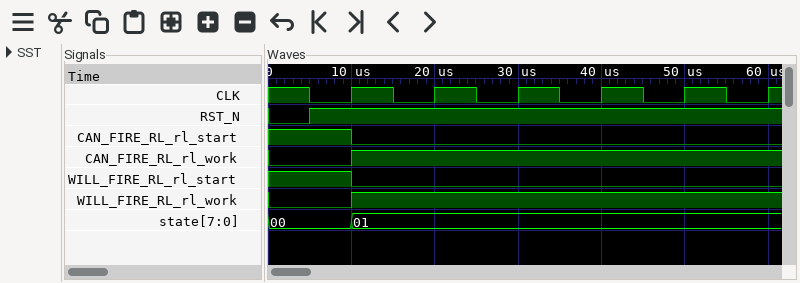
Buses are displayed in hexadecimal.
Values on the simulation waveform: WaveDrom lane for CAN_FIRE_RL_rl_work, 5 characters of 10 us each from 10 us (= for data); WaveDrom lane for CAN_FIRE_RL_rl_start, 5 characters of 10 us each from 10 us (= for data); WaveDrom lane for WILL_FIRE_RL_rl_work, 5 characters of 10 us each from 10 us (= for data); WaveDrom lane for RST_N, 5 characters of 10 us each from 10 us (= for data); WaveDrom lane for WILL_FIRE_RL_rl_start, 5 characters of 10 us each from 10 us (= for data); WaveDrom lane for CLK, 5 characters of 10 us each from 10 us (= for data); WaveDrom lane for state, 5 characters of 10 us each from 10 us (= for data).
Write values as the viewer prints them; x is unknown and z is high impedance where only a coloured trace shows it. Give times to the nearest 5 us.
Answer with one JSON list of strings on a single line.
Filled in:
["{name: 'CAN_FIRE_RL_rl_work', wave: '1....'}", "{name: 'CAN_FIRE_RL_rl_start', wave: '0....'}", "{name: 'WILL_FIRE_RL_rl_work', wave: '1....'}", "{name: 'RST_N', wave: '1....'}", "{name: 'WILL_FIRE_RL_rl_start', wave: '0....'}", "{name: 'CLK', wave: 'p....'}", "{name: 'state', wave: '=....', data: '01'}"]
